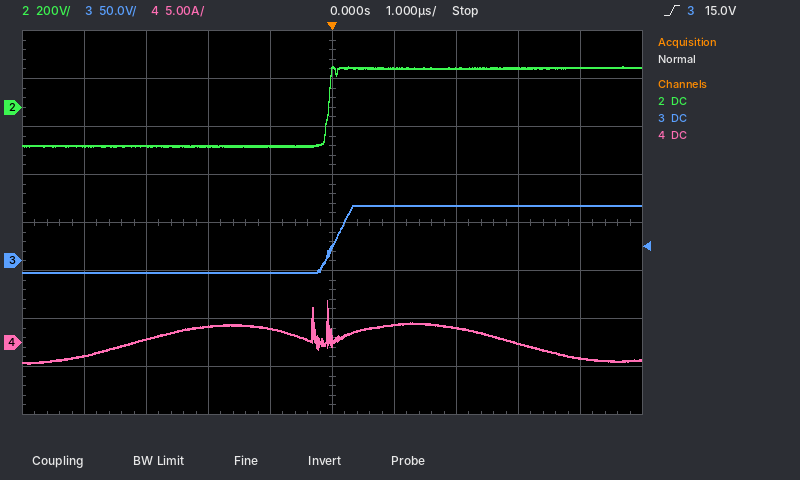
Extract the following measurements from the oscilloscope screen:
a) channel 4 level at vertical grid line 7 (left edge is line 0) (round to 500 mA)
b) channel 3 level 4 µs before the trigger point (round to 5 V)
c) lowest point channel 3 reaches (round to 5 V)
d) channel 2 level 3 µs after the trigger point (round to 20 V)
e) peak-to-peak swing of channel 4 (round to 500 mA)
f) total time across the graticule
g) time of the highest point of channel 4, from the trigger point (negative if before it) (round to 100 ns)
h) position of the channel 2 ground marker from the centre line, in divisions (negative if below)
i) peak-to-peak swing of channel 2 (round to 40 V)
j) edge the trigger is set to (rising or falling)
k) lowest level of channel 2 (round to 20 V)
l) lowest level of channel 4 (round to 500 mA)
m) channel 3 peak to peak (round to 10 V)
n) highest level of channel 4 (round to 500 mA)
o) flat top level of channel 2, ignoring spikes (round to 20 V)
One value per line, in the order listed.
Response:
1.5 A
-10 V
-10 V
160 V
6.5 A
10 µs
-100 ns
+2.4 div
320 V
rising
-160 V
-2.0 A
70 V
4.5 A
160 V
